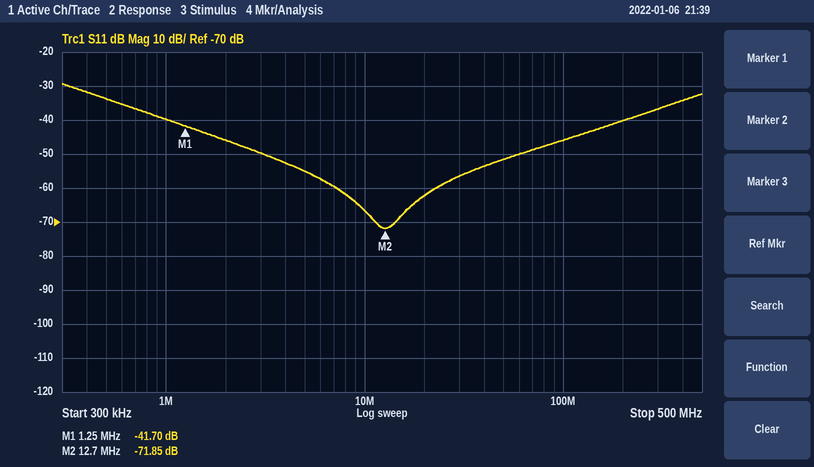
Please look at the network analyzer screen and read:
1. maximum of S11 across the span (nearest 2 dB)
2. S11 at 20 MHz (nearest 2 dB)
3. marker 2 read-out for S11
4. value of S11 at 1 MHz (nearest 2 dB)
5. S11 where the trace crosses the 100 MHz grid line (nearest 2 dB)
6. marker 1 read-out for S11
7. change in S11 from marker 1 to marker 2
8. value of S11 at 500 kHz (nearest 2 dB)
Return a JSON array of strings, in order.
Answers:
["-30 dB", "-62 dB", "-71.85 dB", "-40 dB", "-46 dB", "-41.70 dB", "-30.15 dB", "-34 dB"]
